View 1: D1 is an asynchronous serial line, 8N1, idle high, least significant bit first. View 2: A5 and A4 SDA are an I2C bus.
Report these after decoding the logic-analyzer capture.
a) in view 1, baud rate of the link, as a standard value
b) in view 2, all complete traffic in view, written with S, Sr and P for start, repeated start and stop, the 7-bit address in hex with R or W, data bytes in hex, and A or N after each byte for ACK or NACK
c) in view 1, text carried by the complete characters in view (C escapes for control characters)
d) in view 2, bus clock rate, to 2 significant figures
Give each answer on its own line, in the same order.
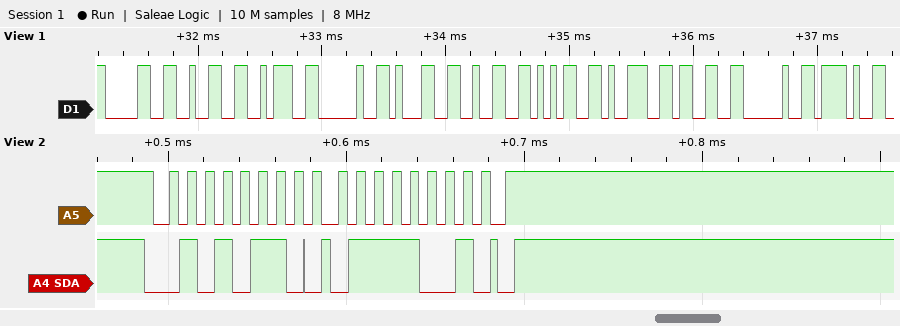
19200 baud
S 2BW A 79 A P
"02: 12593 /"
100 kHz
